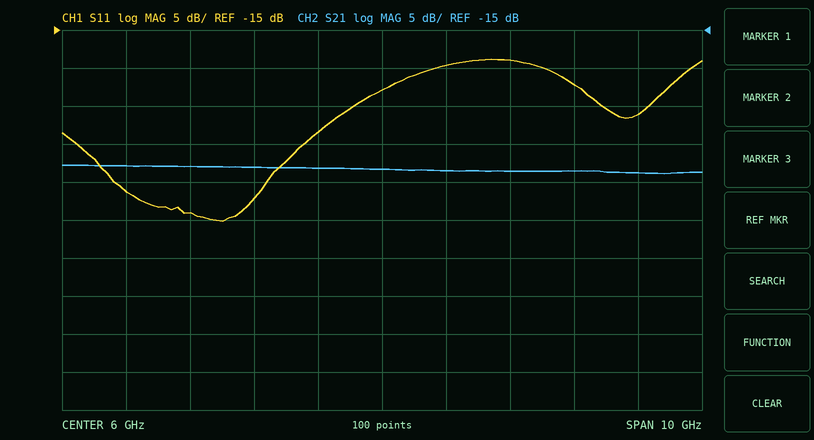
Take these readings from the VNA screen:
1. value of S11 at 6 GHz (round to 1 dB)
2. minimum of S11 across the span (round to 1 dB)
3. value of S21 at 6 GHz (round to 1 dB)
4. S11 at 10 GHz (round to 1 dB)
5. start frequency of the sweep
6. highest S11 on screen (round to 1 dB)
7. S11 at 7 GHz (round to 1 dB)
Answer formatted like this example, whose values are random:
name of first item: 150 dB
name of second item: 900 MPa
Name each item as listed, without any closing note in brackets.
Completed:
value of S11 at 6 GHz: -23 dB
minimum of S11 across the span: -40 dB
value of S21 at 6 GHz: -33 dB
S11 at 10 GHz: -26 dB
start frequency of the sweep: 1 GHz
highest S11 on screen: -19 dB
S11 at 7 GHz: -20 dB
